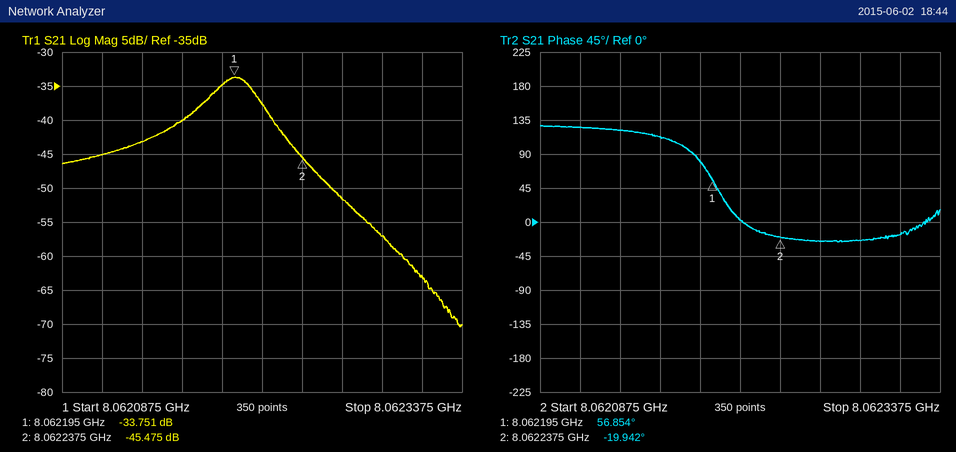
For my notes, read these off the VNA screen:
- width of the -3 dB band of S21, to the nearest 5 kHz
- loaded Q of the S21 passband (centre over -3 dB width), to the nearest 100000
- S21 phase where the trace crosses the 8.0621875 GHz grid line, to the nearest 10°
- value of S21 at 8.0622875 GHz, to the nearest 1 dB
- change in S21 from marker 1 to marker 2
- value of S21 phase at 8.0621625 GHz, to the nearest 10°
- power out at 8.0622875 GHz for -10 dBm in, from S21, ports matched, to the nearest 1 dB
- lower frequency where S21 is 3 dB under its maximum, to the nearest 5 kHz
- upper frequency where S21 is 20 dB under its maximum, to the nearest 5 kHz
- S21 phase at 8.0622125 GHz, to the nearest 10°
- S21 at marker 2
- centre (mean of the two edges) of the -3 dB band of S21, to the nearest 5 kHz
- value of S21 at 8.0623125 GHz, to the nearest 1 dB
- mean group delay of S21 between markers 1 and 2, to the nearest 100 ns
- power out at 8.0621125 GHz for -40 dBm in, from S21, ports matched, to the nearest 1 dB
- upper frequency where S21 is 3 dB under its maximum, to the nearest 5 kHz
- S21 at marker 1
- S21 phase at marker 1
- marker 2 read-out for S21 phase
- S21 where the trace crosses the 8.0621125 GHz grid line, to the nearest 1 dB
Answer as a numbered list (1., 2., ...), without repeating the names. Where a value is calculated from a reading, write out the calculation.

1. 8.062210 GHz − 8.062180 GHz = 30 kHz
2. 8.0622 GHz / 30 kHz ≈ 268740, so 300000 to the nearest 100000
3. 80°
4. -57 dB
5. -45.475 − (-33.751) = -11.724 dB
6. 110°
7. -10 dBm + (-57 dB) = -67 dBm
8. 8.062180 GHz
9. 8.062270 GHz
10. 0°
11. -45.475 dB
12. 8.062195 GHz
13. -63 dB
14. −(-19.942° − (56.854°))/(360° × 42.5 kHz) ≈ 5.0 µs
15. -40 dBm + (-45 dB) = -85 dBm
16. 8.062210 GHz
17. -33.751 dB
18. 56.854°
19. -19.942°
20. -45 dB
